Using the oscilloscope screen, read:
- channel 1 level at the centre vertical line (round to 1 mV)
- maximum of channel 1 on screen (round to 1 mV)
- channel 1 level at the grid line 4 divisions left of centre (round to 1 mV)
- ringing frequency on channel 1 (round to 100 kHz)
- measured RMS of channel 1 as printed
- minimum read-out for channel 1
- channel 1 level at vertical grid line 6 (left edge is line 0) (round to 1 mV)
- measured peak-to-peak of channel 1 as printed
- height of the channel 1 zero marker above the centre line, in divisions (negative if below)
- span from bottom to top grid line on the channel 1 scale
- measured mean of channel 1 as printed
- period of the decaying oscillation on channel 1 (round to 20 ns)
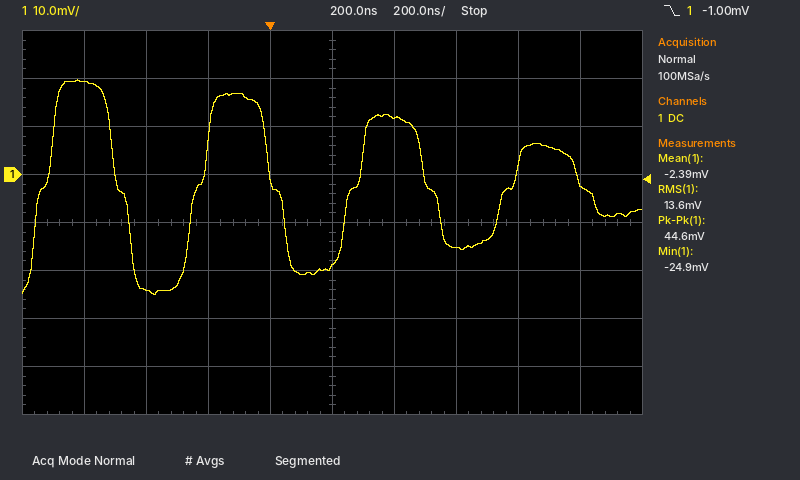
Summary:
-19 mV
20 mV
19 mV
2.0 MHz
13.6 mV
-24.9 mV
12 mV
44.6 mV
+1.0 div
80 mV
-2.39 mV
500 ns
